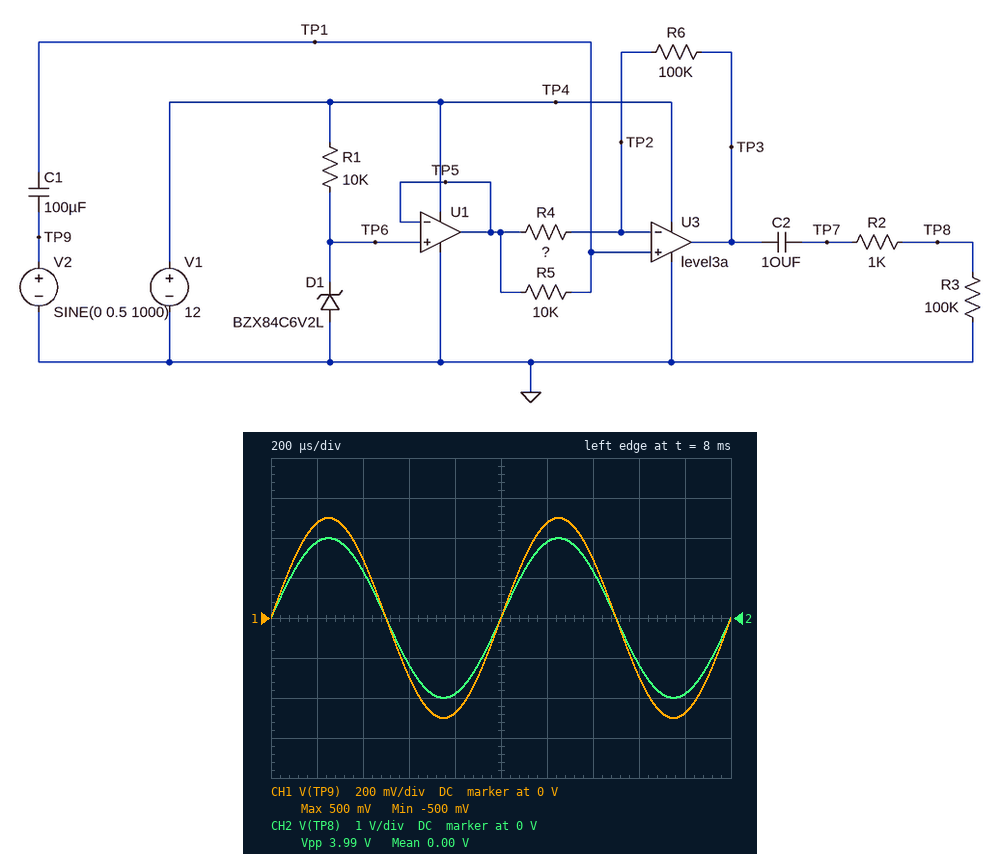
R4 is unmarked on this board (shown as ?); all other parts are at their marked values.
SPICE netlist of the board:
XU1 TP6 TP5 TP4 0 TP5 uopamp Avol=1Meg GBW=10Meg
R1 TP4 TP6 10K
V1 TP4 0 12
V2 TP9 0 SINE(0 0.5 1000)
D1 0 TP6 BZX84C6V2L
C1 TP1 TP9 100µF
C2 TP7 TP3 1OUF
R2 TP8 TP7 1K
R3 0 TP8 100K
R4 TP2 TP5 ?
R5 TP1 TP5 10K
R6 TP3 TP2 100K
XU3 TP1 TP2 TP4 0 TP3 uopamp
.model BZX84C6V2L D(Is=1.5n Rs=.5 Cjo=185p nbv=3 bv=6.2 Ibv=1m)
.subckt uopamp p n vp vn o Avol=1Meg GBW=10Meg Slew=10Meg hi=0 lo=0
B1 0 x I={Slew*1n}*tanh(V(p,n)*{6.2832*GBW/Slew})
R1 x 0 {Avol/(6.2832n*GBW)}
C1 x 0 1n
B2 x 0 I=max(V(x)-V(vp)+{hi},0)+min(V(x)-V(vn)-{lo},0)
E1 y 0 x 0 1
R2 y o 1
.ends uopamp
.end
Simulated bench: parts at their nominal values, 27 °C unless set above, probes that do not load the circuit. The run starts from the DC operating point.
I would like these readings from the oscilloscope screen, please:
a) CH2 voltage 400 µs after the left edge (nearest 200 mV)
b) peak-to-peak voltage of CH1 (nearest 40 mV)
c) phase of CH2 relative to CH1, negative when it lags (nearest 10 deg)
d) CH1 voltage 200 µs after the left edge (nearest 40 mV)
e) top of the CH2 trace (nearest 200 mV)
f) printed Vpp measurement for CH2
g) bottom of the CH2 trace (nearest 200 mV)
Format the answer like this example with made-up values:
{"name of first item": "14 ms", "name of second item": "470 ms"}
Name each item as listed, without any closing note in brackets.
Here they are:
{"CH2 voltage 400 µs after the left edge": "1.2 V", "peak-to-peak voltage of CH1": "1.00 V", "phase of CH2 relative to CH1, negative when it lags": "0 deg", "CH1 voltage 200 µs after the left edge": "480 mV", "top of the CH2 trace": "2.0 V", "printed Vpp measurement for CH2": "3.99 V", "bottom of the CH2 trace": "-2.0 V"}
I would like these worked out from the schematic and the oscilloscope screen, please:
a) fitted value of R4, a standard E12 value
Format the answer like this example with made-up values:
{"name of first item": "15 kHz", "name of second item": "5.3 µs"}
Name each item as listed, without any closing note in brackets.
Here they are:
{"fitted value of R4, a standard E12 value": "33 kΩ"}
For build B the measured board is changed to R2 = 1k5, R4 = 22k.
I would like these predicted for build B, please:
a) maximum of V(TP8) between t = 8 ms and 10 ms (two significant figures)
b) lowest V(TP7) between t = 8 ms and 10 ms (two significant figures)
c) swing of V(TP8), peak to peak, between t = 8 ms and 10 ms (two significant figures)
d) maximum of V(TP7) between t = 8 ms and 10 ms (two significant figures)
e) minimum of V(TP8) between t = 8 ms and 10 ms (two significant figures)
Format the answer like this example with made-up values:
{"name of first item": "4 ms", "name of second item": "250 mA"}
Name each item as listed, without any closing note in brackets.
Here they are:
{"maximum of V(TP8) between t = 8 ms and 10 ms": "2.7 V", "lowest V(TP7) between t = 8 ms and 10 ms": "-2.8 V", "swing of V(TP8), peak to peak, between t = 8 ms and 10 ms": "5.5 V", "maximum of V(TP7) between t = 8 ms and 10 ms": "2.8 V", "minimum of V(TP8) between t = 8 ms and 10 ms": "-2.7 V"}
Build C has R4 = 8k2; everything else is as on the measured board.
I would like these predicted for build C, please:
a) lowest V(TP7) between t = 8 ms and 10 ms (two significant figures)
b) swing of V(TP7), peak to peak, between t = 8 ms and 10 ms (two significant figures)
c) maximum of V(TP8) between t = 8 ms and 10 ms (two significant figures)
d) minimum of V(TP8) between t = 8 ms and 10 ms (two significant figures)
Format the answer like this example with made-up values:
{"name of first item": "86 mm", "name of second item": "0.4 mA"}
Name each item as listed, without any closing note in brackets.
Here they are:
{"lowest V(TP7) between t = 8 ms and 10 ms": "-6.2 V", "swing of V(TP7), peak to peak, between t = 8 ms and 10 ms": "12 V", "maximum of V(TP8) between t = 8 ms and 10 ms": "5.8 V", "minimum of V(TP8) between t = 8 ms and 10 ms": "-6.1 V"}
